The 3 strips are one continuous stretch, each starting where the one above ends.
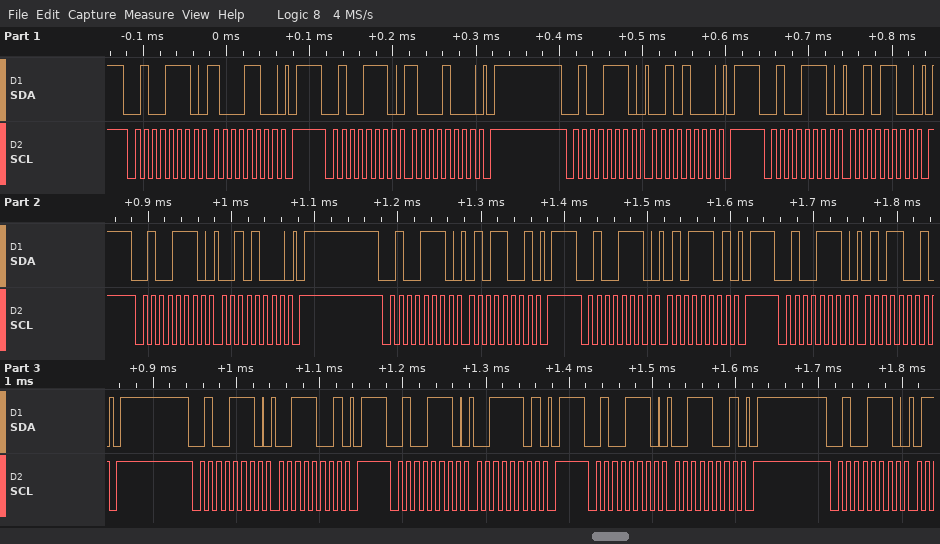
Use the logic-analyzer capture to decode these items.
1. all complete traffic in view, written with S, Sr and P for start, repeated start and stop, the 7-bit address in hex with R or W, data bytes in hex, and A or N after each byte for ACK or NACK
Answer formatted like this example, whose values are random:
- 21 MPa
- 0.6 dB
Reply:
- S 27W A 8C A P S 27W A 88 A P S 27W A 28 A P S 27W A 2C A P S 27W A 28 A P S 27W A 59 A P S 27W A 5D A P S 27W A 59 A P S 27W A 39 A P S 27W A 3D A P S 27W A 39 A P S 27W A
